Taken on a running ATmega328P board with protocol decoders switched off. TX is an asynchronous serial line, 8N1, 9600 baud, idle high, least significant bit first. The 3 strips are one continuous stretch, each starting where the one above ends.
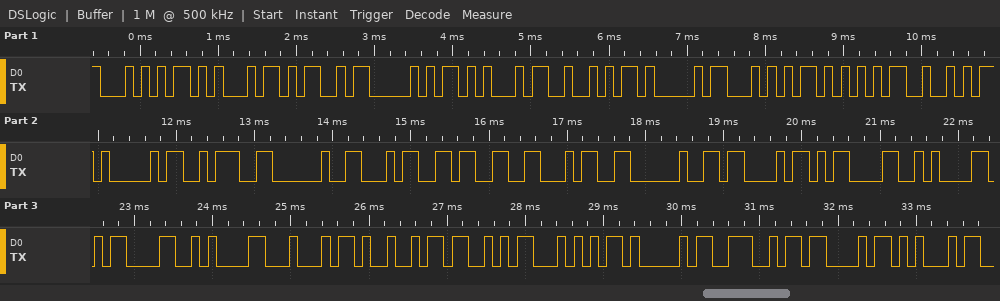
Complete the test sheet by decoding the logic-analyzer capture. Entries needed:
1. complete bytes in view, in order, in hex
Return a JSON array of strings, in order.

["0x54 0x45 0x4D 0x50 0x45 0x52 0x41 0x54 0x55 0x52 0x41 0x3A 0x20 0x34 0x33 0x34 0x20 0x43 0x0D 0x0A 0x0D 0x0A 0x44 0x49 0x53 0x54 0x41 0x4E 0x43 0x45"]
